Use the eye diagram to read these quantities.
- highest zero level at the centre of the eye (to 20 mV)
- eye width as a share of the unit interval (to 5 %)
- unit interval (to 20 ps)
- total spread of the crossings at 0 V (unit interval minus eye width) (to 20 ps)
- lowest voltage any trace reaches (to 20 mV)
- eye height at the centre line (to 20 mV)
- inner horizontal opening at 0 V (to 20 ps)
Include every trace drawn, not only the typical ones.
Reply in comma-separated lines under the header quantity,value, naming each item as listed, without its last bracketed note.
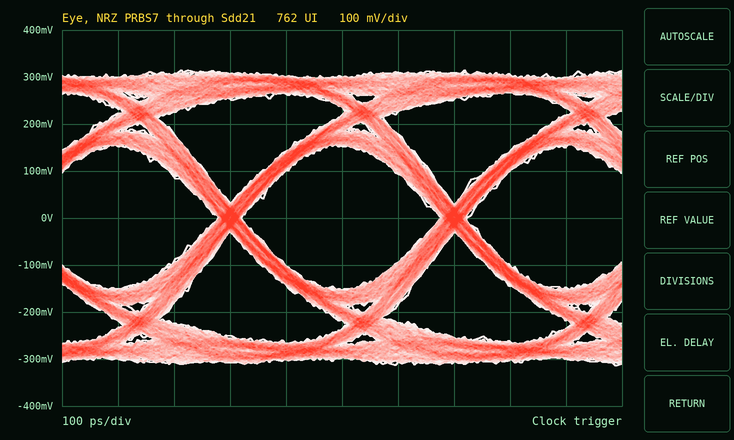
quantity,value
highest zero level at the centre of the eye,-160 mV
eye width as a share of the unit interval,90 %
unit interval,400 ps
total spread of the crossings at 0 V (unit interval minus eye width),40 ps
lowest voltage any trace reaches,-320 mV
eye height at the centre line,300 mV
inner horizontal opening at 0 V,360 ps
